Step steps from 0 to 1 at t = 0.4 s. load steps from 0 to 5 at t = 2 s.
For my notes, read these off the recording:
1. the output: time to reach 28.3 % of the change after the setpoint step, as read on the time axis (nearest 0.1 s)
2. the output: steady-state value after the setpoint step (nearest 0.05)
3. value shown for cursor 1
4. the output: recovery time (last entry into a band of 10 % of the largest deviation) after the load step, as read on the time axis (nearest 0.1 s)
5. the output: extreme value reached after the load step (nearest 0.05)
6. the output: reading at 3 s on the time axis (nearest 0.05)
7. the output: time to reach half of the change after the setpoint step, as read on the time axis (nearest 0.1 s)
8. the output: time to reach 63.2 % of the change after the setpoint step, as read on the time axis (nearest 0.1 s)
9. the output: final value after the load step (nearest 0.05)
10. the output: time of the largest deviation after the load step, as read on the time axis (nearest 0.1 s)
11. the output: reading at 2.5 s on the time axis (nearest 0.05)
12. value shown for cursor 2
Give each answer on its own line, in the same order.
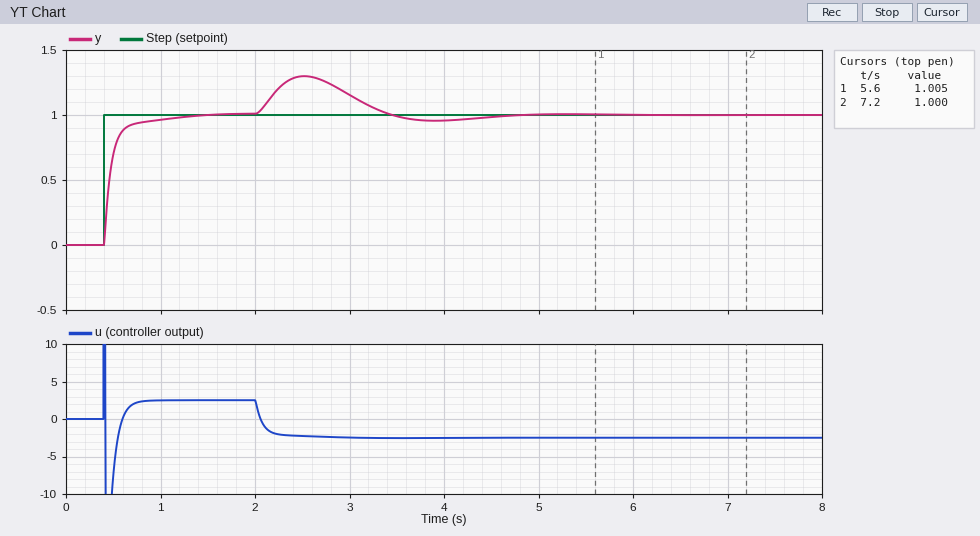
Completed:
0.4 s
1.00
1.005
4.3 s
1.30
1.15
0.5 s
0.5 s
1.00
2.5 s
1.30
1.000
